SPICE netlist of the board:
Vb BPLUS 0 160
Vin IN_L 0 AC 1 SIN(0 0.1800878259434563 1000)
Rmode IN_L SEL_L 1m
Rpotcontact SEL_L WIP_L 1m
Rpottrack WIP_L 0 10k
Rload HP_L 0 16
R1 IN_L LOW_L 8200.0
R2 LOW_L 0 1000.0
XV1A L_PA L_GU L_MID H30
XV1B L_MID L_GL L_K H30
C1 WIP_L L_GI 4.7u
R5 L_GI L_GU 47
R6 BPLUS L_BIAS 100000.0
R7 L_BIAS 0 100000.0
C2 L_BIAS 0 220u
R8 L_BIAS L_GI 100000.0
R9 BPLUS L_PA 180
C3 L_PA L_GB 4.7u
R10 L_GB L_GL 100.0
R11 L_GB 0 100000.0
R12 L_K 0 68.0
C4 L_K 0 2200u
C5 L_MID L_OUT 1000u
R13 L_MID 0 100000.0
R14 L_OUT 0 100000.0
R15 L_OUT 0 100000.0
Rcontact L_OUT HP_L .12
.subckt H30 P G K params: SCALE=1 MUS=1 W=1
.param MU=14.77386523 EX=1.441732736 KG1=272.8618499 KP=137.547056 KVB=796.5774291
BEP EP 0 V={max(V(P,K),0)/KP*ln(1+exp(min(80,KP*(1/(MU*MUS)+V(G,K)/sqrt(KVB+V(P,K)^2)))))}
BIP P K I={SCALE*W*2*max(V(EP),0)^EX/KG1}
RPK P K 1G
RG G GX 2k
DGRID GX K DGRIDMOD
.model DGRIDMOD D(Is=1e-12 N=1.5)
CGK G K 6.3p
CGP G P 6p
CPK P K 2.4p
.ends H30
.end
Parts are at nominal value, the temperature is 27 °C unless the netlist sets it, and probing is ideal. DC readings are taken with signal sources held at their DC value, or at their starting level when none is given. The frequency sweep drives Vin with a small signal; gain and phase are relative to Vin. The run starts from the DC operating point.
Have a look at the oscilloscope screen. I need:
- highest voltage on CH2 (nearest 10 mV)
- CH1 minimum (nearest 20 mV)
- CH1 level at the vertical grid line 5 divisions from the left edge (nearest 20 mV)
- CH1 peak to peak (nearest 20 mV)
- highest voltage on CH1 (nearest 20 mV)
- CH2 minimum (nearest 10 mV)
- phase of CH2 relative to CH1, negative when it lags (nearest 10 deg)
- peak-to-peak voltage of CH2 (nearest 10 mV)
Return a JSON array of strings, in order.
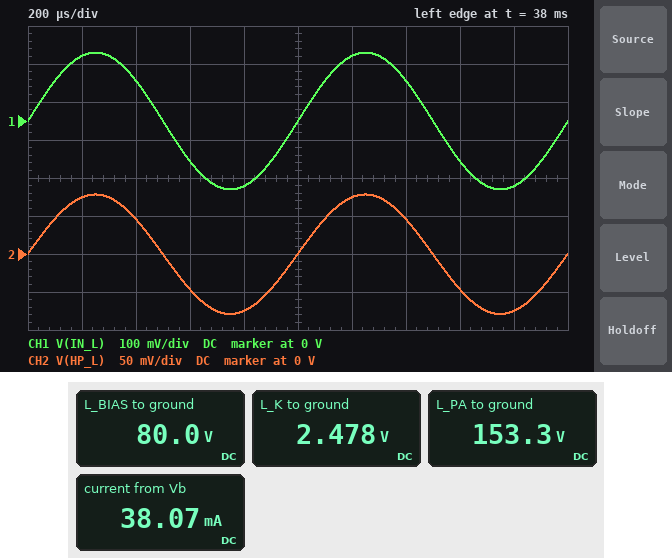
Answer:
["80 mV", "-180 mV", "0 V", "360 mV", "180 mV", "-80 mV", "0 deg", "160 mV"]
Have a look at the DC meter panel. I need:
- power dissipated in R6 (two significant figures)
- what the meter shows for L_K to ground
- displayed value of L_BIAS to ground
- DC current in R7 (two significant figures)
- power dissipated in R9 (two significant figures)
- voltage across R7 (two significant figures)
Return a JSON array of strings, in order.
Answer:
["64 mW", "2.478 V", "80.0 V", "800 µA", "250 mW", "80 V"]
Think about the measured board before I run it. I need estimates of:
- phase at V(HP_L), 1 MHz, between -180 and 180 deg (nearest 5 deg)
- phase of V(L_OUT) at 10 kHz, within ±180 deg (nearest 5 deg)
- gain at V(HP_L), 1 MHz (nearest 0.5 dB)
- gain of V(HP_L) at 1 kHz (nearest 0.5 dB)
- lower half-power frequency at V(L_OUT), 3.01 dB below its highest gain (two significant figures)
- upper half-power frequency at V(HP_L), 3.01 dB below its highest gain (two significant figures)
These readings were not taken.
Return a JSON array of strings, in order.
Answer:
["0 deg", "0 deg", "-7.0 dB", "-7.0 dB", "5.5 Hz", "47 MHz"]
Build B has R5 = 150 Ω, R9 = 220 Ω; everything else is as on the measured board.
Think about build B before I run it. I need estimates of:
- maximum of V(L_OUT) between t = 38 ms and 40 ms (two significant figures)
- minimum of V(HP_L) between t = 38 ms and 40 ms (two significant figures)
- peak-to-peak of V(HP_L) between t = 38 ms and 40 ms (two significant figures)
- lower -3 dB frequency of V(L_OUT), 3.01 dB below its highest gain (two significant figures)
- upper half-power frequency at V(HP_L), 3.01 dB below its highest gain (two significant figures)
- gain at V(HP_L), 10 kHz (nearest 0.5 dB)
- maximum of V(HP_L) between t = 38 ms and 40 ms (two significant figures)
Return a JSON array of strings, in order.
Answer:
["84 mV", "-84 mV", "170 mV", "5.7 Hz", "33 MHz", "-6.5 dB", "83 mV"]
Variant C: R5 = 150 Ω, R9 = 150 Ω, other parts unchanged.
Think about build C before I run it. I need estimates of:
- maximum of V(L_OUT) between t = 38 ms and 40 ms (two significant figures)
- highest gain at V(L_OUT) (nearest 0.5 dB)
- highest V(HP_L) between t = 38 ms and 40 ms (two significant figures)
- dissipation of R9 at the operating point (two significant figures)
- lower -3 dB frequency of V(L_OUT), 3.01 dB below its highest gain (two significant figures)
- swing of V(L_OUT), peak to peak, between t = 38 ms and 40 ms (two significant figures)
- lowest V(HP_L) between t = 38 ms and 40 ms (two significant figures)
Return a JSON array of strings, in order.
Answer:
["75 mV", "-7.5 dB", "74 mV", "210 mW", "5.2 Hz", "150 mV", "-75 mV"]
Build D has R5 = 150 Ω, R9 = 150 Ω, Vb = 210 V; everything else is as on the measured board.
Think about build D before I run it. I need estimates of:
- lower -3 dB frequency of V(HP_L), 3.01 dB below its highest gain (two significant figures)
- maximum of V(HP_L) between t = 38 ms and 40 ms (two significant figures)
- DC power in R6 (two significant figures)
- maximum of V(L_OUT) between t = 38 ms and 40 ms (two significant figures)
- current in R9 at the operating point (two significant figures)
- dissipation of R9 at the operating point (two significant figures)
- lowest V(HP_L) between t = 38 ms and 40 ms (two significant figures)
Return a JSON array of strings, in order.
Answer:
["5.7 Hz", "82 mV", "110 mW", "83 mV", "51 mA", "390 mW", "-83 mV"]
